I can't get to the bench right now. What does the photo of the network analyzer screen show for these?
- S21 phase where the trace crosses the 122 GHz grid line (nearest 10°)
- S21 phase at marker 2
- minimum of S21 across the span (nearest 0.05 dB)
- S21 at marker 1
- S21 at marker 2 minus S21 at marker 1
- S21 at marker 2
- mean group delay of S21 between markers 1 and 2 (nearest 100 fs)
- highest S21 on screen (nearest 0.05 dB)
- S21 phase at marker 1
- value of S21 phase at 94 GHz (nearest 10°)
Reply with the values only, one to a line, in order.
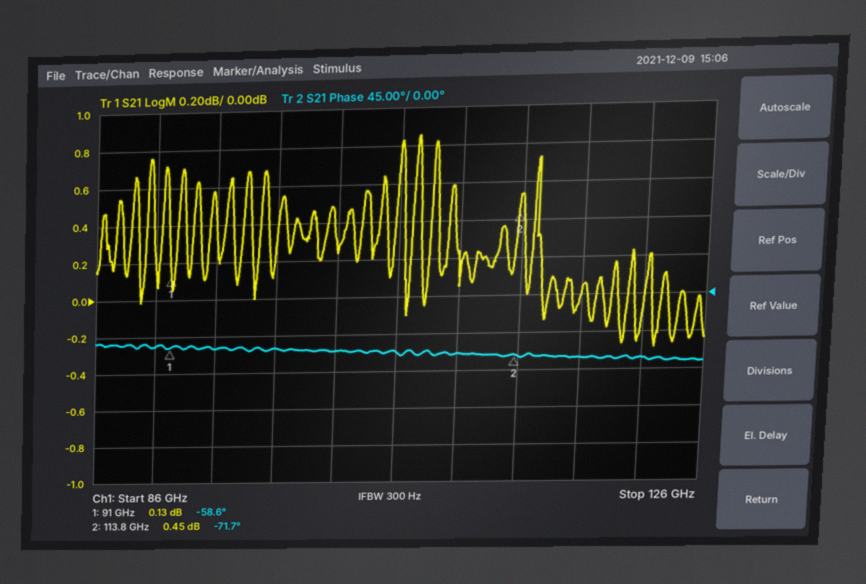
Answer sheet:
-80°
-71.7°
-0.30 dB
0.13 dB
0.32 dB
0.45 dB
1.6 ps
0.85 dB
-58.6°
-60°
